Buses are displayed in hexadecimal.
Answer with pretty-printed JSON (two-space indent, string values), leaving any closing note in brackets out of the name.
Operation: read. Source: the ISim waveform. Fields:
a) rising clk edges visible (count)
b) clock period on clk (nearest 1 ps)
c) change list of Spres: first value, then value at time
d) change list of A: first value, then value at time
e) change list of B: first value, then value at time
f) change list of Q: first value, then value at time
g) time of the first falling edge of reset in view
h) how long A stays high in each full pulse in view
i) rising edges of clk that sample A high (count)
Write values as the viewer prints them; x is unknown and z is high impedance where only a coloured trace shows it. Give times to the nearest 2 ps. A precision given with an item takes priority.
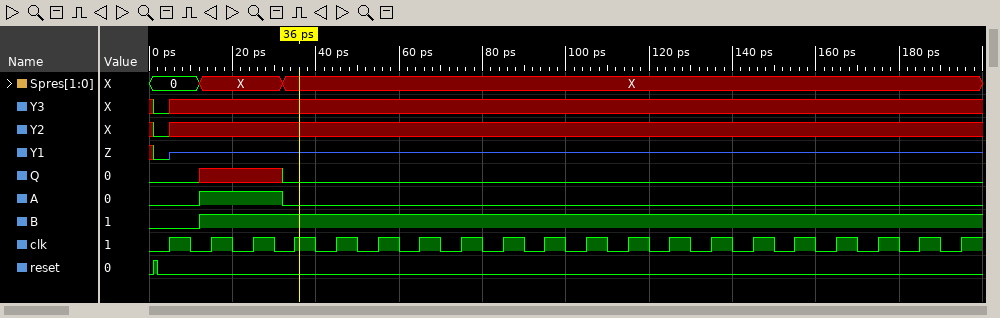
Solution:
{
  "rising clk edges visible": "20",
  "clock period on clk": "10 ps",
  "change list of Spres: first value, then value at time": "0, X at 12 ps, X at 32 ps",
  "change list of A: first value, then value at time": "0, 1 at 12 ps, 0 at 32 ps",
  "change list of B: first value, then value at time": "0, 1 at 12 ps",
  "change list of Q: first value, then value at time": "0, x at 12 ps, 0 at 32 ps",
  "time of the first falling edge of reset in view": "2 ps",
  "how long A stays high in each full pulse in view": "20 ps",
  "rising edges of clk that sample A high": "2"
}
